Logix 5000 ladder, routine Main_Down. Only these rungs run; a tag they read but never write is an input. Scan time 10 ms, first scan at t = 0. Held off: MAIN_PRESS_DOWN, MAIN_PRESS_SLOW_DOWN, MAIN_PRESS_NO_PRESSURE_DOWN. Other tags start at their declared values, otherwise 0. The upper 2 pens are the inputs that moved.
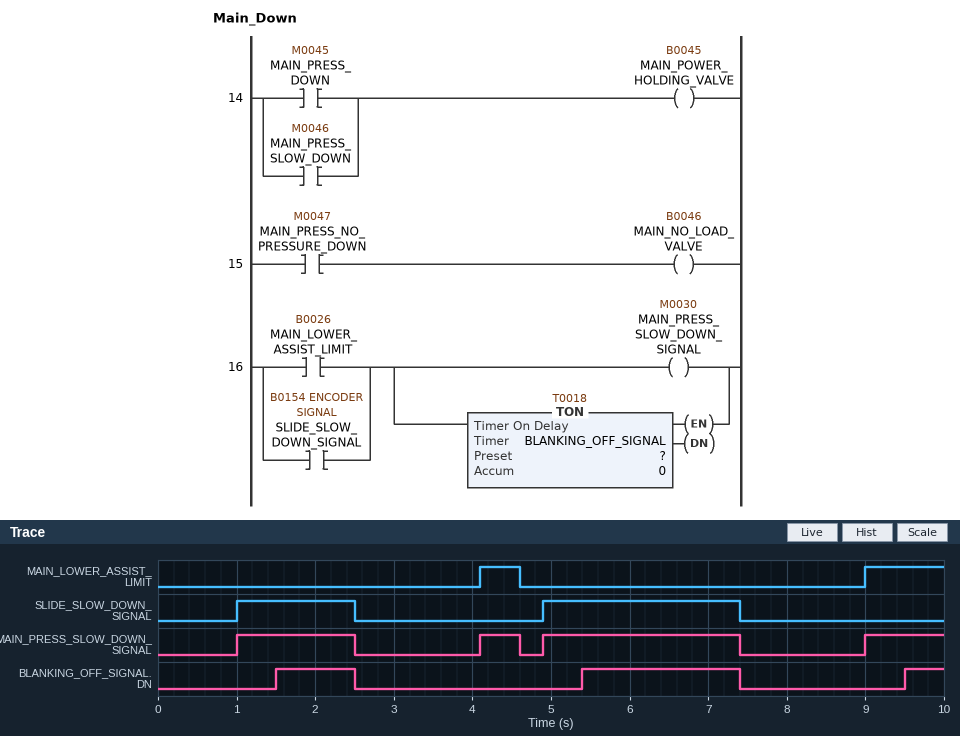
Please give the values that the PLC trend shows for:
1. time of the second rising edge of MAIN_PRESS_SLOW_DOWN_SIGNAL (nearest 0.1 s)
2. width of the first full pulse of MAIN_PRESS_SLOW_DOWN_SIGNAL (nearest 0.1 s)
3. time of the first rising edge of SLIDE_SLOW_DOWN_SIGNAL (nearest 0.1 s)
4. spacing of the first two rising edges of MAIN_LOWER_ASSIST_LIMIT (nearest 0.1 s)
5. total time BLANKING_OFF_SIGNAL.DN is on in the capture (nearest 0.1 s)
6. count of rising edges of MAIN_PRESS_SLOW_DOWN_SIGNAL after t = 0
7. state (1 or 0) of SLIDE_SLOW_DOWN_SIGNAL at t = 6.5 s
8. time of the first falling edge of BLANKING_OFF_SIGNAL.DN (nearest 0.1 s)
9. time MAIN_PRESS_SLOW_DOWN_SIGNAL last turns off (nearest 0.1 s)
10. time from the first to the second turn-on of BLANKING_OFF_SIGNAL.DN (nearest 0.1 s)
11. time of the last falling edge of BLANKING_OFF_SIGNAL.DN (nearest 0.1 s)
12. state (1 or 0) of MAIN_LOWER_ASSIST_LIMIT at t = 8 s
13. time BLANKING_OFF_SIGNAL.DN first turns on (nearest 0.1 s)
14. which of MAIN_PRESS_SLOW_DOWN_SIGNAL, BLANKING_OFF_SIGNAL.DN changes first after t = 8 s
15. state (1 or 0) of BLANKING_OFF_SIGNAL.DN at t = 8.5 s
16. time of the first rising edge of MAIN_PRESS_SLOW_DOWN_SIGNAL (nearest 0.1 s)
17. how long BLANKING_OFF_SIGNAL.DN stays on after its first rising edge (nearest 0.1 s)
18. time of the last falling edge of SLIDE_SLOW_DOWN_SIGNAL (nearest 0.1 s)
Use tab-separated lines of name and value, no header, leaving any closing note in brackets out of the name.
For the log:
time of the second rising edge of MAIN_PRESS_SLOW_DOWN_SIGNAL	4.1 s
width of the first full pulse of MAIN_PRESS_SLOW_DOWN_SIGNAL	1.5 s
time of the first rising edge of SLIDE_SLOW_DOWN_SIGNAL	1.0 s
spacing of the first two rising edges of MAIN_LOWER_ASSIST_LIMIT	4.9 s
total time BLANKING_OFF_SIGNAL.DN is on in the capture	3.5 s
count of rising edges of MAIN_PRESS_SLOW_DOWN_SIGNAL after t = 0	4
state (1 or 0) of SLIDE_SLOW_DOWN_SIGNAL at t = 6.5 s	1
time of the first falling edge of BLANKING_OFF_SIGNAL.DN	2.5 s
time MAIN_PRESS_SLOW_DOWN_SIGNAL last turns off	7.4 s
time from the first to the second turn-on of BLANKING_OFF_SIGNAL.DN	3.9 s
time of the last falling edge of BLANKING_OFF_SIGNAL.DN	7.4 s
state (1 or 0) of MAIN_LOWER_ASSIST_LIMIT at t = 8 s	0
time BLANKING_OFF_SIGNAL.DN first turns on	1.5 s
which of MAIN_PRESS_SLOW_DOWN_SIGNAL, BLANKING_OFF_SIGNAL.DN changes first after t = 8 s	MAIN_PRESS_SLOW_DOWN_SIGNAL
state (1 or 0) of BLANKING_OFF_SIGNAL.DN at t = 8.5 s	0
time of the first rising edge of MAIN_PRESS_SLOW_DOWN_SIGNAL	1.0 s
how long BLANKING_OFF_SIGNAL.DN stays on after its first rising edge	1.0 s
time of the last falling edge of SLIDE_SLOW_DOWN_SIGNAL	7.4 s
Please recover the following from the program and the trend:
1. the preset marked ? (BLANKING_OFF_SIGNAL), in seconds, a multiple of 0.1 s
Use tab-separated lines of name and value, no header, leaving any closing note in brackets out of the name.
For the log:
the preset marked ? (BLANKING_OFF_SIGNAL), in seconds, a multiple of 0.1 s	0.5 s
